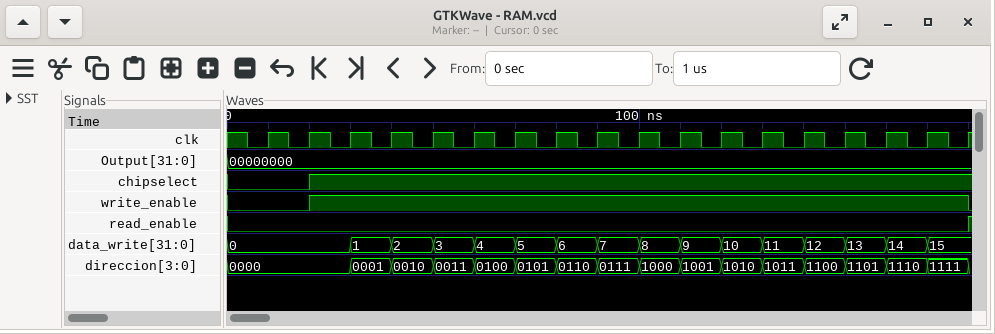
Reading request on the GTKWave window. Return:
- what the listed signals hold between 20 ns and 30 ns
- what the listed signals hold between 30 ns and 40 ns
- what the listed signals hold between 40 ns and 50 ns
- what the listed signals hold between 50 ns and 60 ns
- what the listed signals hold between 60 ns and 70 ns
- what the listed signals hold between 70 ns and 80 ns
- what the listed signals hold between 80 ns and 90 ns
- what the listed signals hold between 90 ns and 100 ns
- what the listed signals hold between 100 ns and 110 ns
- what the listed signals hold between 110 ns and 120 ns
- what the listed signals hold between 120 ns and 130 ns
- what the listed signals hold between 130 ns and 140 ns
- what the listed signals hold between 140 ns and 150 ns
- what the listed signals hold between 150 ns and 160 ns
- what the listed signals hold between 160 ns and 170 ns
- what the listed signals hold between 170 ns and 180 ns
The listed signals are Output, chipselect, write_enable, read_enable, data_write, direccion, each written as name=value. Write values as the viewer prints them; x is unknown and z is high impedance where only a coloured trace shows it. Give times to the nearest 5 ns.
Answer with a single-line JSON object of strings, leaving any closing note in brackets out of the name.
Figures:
{"what the listed signals hold between 20 ns and 30 ns": "Output=00000000, chipselect=1, write_enable=1, read_enable=0, data_write=0, direccion=0000", "what the listed signals hold between 30 ns and 40 ns": "Output=00000000, chipselect=1, write_enable=1, read_enable=0, data_write=1, direccion=0001", "what the listed signals hold between 40 ns and 50 ns": "Output=00000000, chipselect=1, write_enable=1, read_enable=0, data_write=2, direccion=0010", "what the listed signals hold between 50 ns and 60 ns": "Output=00000000, chipselect=1, write_enable=1, read_enable=0, data_write=3, direccion=0011", "what the listed signals hold between 60 ns and 70 ns": "Output=00000000, chipselect=1, write_enable=1, read_enable=0, data_write=4, direccion=0100", "what the listed signals hold between 70 ns and 80 ns": "Output=00000000, chipselect=1, write_enable=1, read_enable=0, data_write=5, direccion=0101", "what the listed signals hold between 80 ns and 90 ns": "Output=00000000, chipselect=1, write_enable=1, read_enable=0, data_write=6, direccion=0110", "what the listed signals hold between 90 ns and 100 ns": "Output=00000000, chipselect=1, write_enable=1, read_enable=0, data_write=7, direccion=0111", "what the listed signals hold between 100 ns and 110 ns": "Output=00000000, chipselect=1, write_enable=1, read_enable=0, data_write=8, direccion=1000", "what the listed signals hold between 110 ns and 120 ns": "Output=00000000, chipselect=1, write_enable=1, read_enable=0, data_write=9, direccion=1001", "what the listed signals hold between 120 ns and 130 ns": "Output=00000000, chipselect=1, write_enable=1, read_enable=0, data_write=10, direccion=1010", "what the listed signals hold between 130 ns and 140 ns": "Output=00000000, chipselect=1, write_enable=1, read_enable=0, data_write=11, direccion=1011", "what the listed signals hold between 140 ns and 150 ns": "Output=00000000, chipselect=1, write_enable=1, read_enable=0, data_write=12, direccion=1100", "what the listed signals hold between 150 ns and 160 ns": "Output=00000000, chipselect=1, write_enable=1, read_enable=0, data_write=13, direccion=1101", "what the listed signals hold between 160 ns and 170 ns": "Output=00000000, chipselect=1, write_enable=1, read_enable=0, data_write=14, direccion=1110", "what the listed signals hold between 170 ns and 180 ns": "Output=00000000, chipselect=1, write_enable=1, read_enable=0, data_write=15, direccion=1111"}
